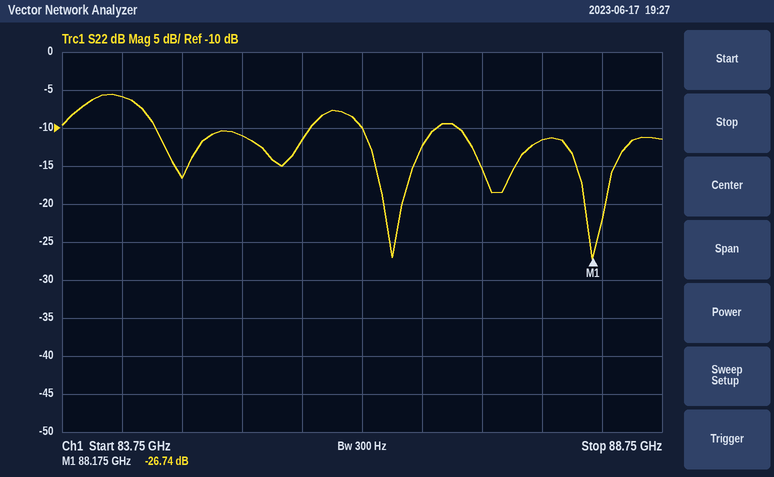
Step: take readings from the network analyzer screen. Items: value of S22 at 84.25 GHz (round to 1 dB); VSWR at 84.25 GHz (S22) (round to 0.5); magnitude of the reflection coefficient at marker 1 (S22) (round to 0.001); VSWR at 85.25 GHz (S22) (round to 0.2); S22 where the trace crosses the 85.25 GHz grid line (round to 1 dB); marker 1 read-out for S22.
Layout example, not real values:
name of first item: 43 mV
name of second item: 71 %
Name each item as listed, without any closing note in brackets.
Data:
value of S22 at 84.25 GHz: -6 dB
VSWR at 84.25 GHz (S22): 3.0
magnitude of the reflection coefficient at marker 1 (S22): 0.046
VSWR at 85.25 GHz (S22): 1.8
S22 where the trace crosses the 85.25 GHz grid line: -11 dB
marker 1 read-out for S22: -26.74 dB
